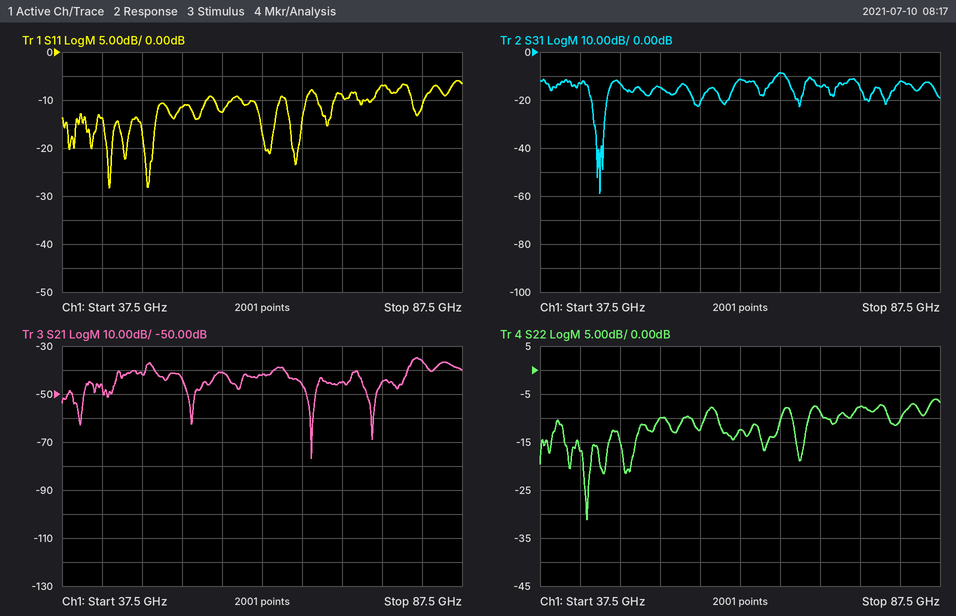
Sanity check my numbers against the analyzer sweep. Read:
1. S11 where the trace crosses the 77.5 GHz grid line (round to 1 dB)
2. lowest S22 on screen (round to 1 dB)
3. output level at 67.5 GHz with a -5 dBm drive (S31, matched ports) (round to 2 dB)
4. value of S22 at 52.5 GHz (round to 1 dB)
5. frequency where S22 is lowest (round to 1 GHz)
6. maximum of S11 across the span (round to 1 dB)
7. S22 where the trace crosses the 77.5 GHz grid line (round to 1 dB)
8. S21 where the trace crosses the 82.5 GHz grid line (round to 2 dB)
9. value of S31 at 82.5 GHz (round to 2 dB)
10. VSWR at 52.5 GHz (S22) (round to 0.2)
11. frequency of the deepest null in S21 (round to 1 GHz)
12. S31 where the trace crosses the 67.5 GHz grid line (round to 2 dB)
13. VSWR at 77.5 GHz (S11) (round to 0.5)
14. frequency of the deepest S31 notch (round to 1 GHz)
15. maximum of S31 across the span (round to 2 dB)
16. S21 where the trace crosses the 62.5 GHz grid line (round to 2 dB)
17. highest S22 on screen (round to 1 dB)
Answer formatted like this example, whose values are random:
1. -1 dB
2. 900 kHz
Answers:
1. -7 dB
2. -31 dB
3. -14 dBm
4. -10 dB
5. 43 GHz
6. -6 dB
7. -8 dB
8. -36 dB
9. -12 dB
10. 2.0
11. 69 GHz
12. -8 dB
13. 2.5
14. 45 GHz
15. -8 dB
16. -42 dB
17. -6 dB
